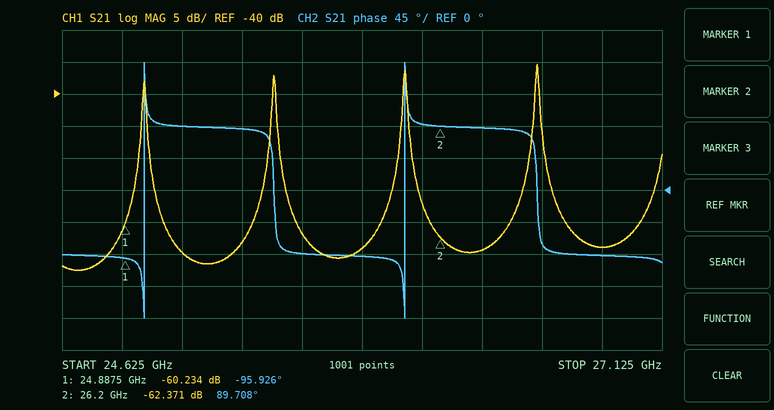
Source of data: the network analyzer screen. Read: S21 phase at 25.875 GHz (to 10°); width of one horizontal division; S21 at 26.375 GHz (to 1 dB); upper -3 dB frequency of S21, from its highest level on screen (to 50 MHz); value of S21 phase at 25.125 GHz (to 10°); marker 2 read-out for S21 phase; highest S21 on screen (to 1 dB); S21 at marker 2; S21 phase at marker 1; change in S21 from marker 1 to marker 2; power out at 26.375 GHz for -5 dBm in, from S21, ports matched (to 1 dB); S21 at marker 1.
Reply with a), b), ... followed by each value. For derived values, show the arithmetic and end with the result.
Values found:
a) -90°
b) 250 MHz
c) -64 dB
d) 26.60 GHz
e) 90°
f) 89.708°
g) -35 dB
h) -62.371 dB
i) -95.926°
j) -62.371 − (-60.234) = -2.137 dB
k) -5 dBm + (-64 dB) = -69 dBm
l) -60.234 dB
